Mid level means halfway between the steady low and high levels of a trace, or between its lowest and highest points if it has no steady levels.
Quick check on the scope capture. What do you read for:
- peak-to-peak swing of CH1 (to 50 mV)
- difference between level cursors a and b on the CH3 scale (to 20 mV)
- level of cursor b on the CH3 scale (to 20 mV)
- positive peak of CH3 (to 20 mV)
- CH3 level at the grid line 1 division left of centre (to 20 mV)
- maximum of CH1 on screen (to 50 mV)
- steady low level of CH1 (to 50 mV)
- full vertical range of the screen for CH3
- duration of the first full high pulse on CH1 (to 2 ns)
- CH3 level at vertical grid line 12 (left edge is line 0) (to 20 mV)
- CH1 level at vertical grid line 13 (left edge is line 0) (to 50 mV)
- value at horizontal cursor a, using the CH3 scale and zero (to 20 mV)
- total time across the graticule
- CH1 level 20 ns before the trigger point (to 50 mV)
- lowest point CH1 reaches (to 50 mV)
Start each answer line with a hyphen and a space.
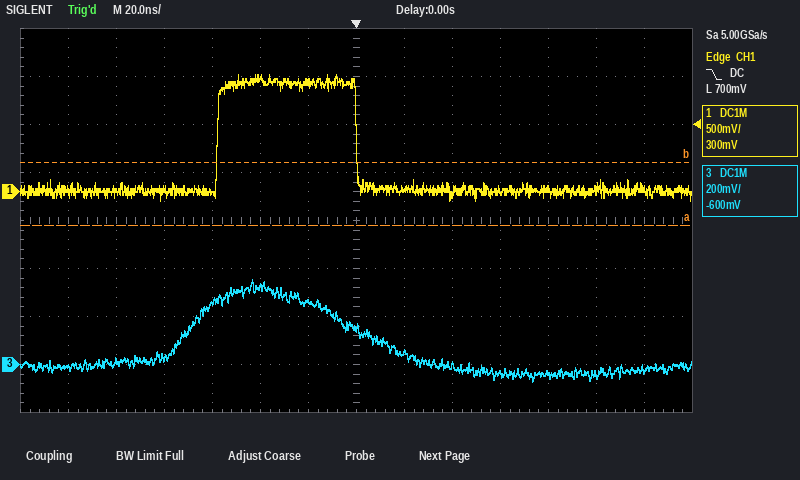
- 1.30 V
- 260 mV
- 840 mV
- 360 mV
- 260 mV
- 1.20 V
- 0 mV
- 1.6 V
- 58 ns
- -40 mV
- 0 mV
- 580 mV
- 280 ns
- 1.15 V
- -100 mV
